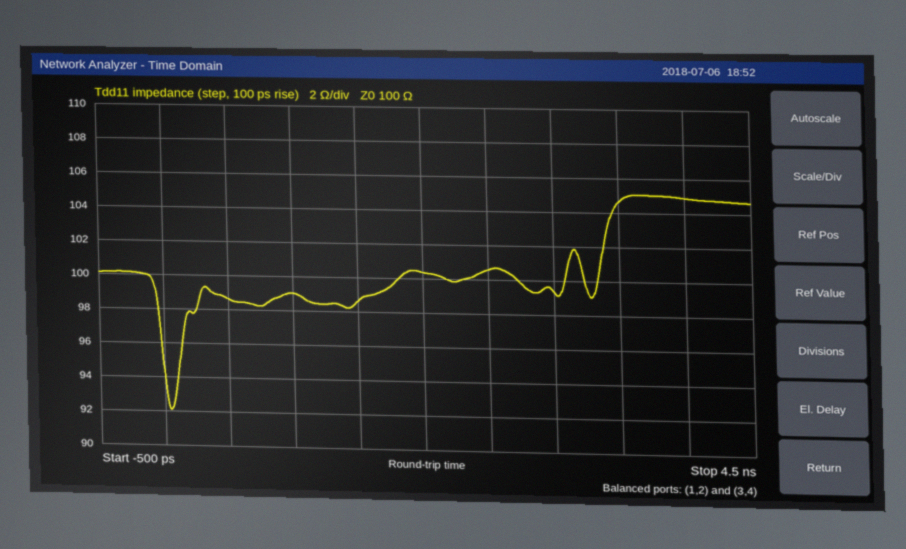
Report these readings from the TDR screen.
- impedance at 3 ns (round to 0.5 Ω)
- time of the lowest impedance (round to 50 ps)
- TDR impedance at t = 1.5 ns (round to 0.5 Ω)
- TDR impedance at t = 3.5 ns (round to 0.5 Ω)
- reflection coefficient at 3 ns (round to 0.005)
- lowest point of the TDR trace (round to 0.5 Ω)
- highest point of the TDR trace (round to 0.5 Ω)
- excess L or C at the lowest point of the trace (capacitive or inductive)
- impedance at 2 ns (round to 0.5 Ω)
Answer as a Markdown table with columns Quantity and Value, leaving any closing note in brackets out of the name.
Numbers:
| Quantity | Value |
|---|---|
| impedance at 3 ns | 99.5 Ω |
| time of the lowest impedance | 50 ps |
| TDR impedance at t = 1.5 ns | 98.5 Ω |
| TDR impedance at t = 3.5 ns | 104.5 Ω |
| reflection coefficient at 3 ns | -0.005 |
| lowest point of the TDR trace | 92.0 Ω |
| highest point of the TDR trace | 105.0 Ω |
| excess L or C at the lowest point of the trace | capacitive |
| impedance at 2 ns | 100.5 Ω |
